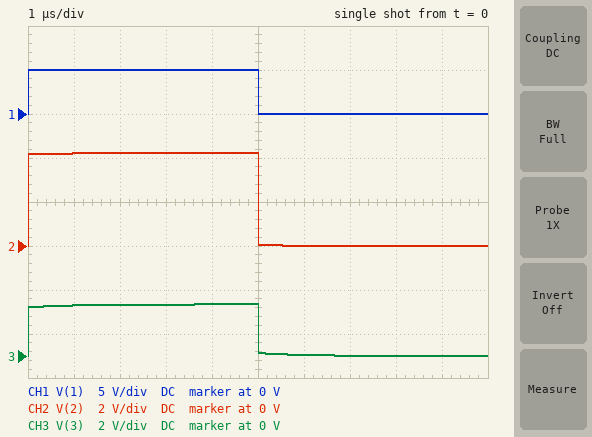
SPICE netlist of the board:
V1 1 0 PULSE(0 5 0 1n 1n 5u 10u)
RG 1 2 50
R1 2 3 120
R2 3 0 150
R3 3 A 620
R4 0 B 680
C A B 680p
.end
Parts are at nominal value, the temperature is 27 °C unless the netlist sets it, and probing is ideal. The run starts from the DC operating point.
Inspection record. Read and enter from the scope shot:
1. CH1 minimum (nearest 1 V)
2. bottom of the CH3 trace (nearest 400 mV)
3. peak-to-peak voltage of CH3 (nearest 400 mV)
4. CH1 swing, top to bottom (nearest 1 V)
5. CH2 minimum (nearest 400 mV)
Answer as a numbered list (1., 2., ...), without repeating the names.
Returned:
1. 0 V
2. 0 V
3. 2.4 V
4. 5 V
5. 0 V
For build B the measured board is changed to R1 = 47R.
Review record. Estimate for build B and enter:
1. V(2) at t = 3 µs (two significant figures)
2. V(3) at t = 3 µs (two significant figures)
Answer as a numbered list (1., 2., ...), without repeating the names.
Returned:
1. 4.0 V
2. 3.0 V
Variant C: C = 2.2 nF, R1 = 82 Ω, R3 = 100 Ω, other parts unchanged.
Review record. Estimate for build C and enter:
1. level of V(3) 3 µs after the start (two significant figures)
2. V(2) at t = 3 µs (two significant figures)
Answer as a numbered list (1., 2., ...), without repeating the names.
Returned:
1. 2.6 V
2. 4.1 V
